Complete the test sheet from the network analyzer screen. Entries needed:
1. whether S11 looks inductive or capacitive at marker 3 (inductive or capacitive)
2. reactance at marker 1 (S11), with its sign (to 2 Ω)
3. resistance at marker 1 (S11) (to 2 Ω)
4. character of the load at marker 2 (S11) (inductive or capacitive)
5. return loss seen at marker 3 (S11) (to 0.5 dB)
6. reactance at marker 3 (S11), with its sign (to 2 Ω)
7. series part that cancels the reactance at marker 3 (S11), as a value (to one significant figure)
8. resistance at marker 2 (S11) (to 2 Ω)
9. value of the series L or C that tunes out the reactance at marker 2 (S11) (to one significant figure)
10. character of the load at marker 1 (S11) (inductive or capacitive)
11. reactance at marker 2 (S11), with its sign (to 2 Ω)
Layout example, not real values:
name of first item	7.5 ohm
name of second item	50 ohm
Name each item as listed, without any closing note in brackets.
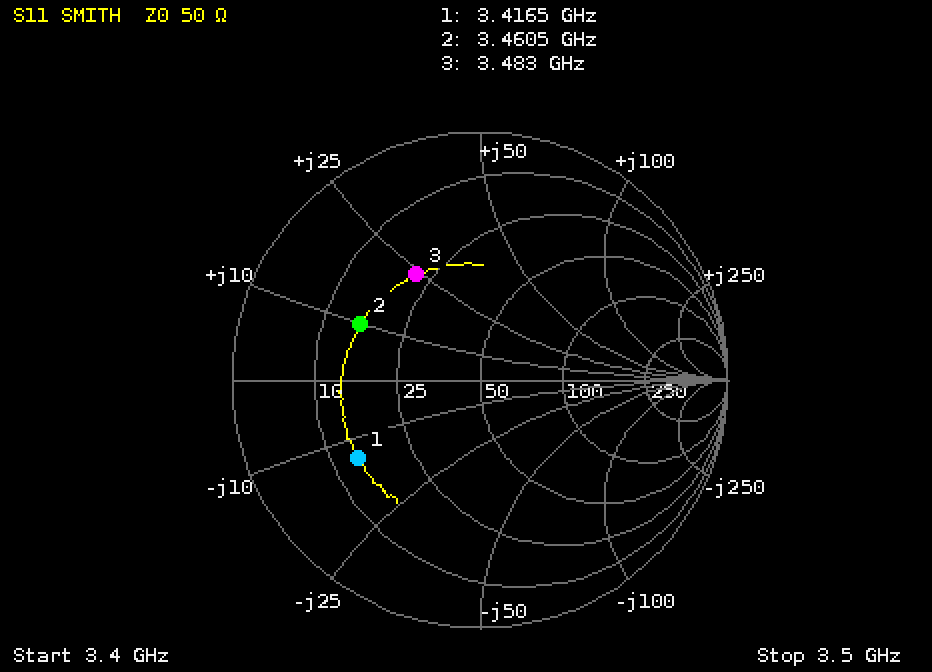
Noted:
whether S11 looks inductive or capacitive at marker 3	inductive
reactance at marker 1 (S11), with its sign	-14 Ω
resistance at marker 1 (S11)	14 Ω
character of the load at marker 2 (S11)	inductive
return loss seen at marker 3 (S11)	6.0 dB
reactance at marker 3 (S11), with its sign	+24 Ω
series part that cancels the reactance at marker 3 (S11), as a value	2 pF
resistance at marker 2 (S11)	16 Ω
value of the series L or C that tunes out the reactance at marker 2 (S11)	5 pF
character of the load at marker 1 (S11)	capacitive
reactance at marker 2 (S11), with its sign	+10 Ω
